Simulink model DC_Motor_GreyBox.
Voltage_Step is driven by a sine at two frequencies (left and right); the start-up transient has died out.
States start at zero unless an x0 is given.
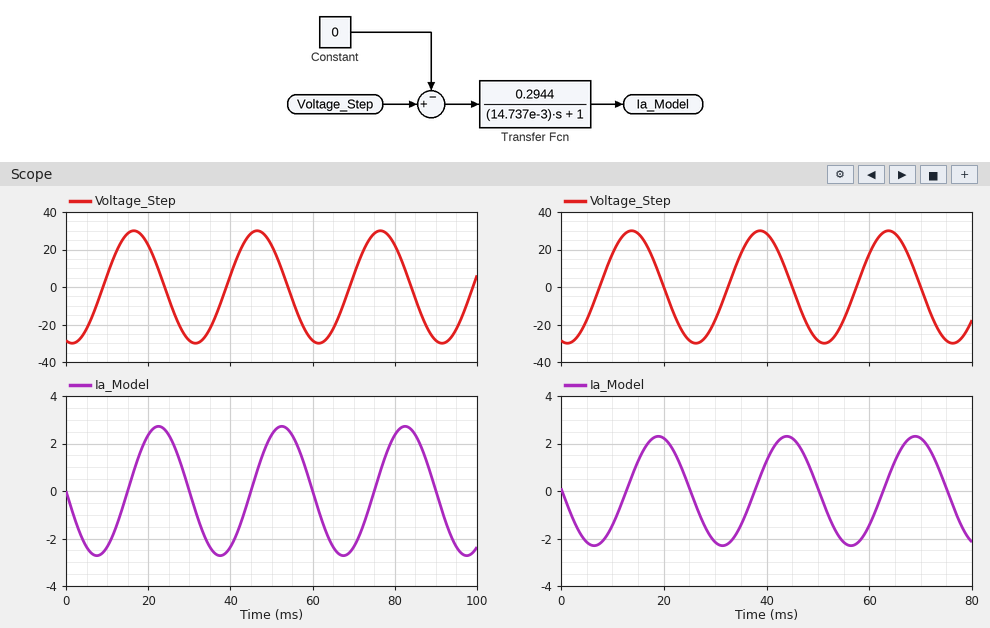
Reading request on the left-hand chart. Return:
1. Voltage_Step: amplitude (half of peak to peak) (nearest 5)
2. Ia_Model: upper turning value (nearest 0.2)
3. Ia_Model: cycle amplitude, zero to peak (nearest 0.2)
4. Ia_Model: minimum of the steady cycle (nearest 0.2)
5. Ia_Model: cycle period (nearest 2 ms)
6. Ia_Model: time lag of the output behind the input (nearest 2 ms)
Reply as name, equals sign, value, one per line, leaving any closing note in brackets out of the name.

Voltage_Step: amplitude (half of peak to peak) = 30
Ia_Model: upper turning value = 2.8
Ia_Model: cycle amplitude, zero to peak = 2.8
Ia_Model: minimum of the steady cycle = -2.8
Ia_Model: cycle period = 30 ms
Ia_Model: time lag of the output behind the input = 6 ms
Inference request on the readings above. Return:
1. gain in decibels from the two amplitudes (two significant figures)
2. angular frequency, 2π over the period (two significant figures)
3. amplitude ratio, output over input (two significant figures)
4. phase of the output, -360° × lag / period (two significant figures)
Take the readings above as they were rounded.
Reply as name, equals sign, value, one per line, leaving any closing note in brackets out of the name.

gain in decibels from the two amplitudes = -21 dB
angular frequency, 2π over the period = 0.21 rad/ms
amplitude ratio, output over input = 0.093
phase of the output, -360° × lag / period = -72°
